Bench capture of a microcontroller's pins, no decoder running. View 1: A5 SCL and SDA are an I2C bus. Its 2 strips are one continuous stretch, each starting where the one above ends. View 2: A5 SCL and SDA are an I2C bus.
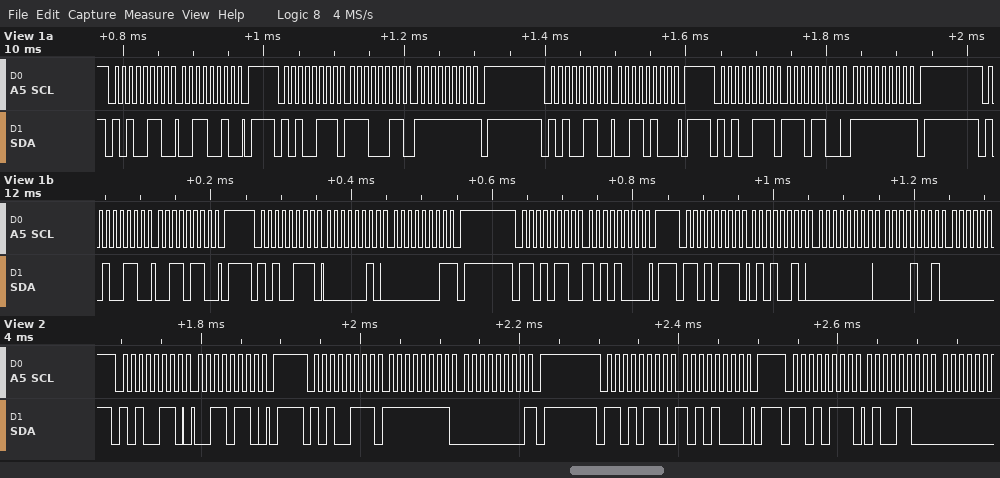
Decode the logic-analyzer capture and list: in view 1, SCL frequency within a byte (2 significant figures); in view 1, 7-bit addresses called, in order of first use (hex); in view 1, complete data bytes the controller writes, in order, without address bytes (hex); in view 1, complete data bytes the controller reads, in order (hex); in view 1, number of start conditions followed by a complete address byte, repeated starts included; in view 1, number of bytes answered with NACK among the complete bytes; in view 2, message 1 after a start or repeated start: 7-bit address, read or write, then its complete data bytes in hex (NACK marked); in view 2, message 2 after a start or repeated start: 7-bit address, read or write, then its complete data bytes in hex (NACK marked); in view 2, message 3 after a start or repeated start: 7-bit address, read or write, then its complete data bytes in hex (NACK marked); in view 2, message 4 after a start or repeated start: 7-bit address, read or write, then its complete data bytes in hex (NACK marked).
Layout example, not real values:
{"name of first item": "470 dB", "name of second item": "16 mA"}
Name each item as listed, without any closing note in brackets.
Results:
{"in view 1, SCL frequency within a byte": "100 kHz", "in view 1, 7-bit addresses called, in order of first use": "0x53 0x6B", "in view 1, complete data bytes the controller writes, in order, without address bytes": "32 34 36 A8", "in view 1, complete data bytes the controller reads, in order": "E3 FF EC FF 02 01 52 00 09", "in view 1, number of start conditions followed by a complete address byte, repeated starts included": "8", "in view 1, number of bytes answered with NACK among the complete bytes": "3", "in view 2, message 1 after a start or repeated start: 7-bit address, read or write, then its complete data bytes in hex": "0x53 write: 36", "in view 2, message 2 after a start or repeated start: 7-bit address, read or write, then its complete data bytes in hex": "0x53 read: FF 00 NACK", "in view 2, message 3 after a start or repeated start: 7-bit address, read or write, then its complete data bytes in hex": "0x6B write: A8", "in view 2, message 4 after a start or repeated start: 7-bit address, read or write, then its complete data bytes in hex": "0x6B read: 4C"}
